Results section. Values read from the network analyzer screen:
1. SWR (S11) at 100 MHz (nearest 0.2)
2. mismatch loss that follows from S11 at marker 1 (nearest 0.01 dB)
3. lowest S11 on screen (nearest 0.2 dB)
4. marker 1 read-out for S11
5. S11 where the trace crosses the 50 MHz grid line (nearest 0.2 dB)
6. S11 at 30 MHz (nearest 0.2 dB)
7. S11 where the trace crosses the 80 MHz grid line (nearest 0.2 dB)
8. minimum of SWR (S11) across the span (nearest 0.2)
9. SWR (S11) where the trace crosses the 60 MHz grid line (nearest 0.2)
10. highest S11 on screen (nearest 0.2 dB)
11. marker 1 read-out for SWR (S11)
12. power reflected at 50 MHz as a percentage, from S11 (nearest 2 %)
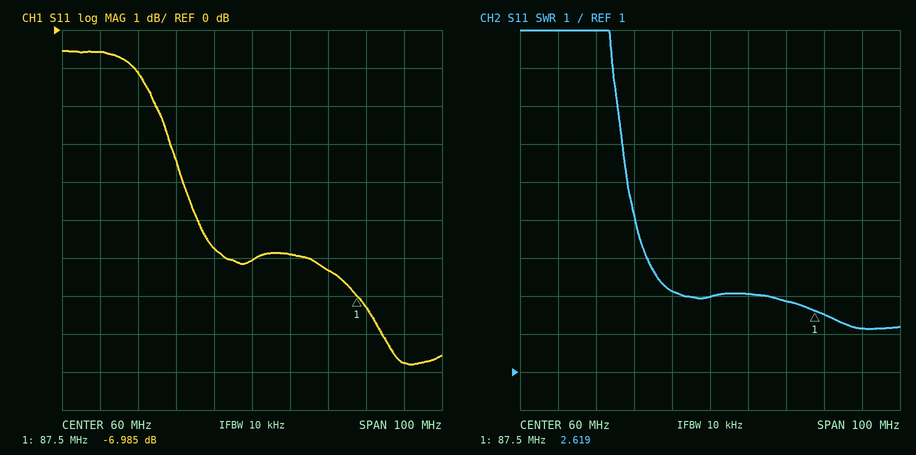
2.2
0.97 dB
-8.8 dB
-6.985 dB
-5.8 dB
-1.2 dB
-6.4 dB
2.2
3.0
-0.6 dB
2.619
26 %
